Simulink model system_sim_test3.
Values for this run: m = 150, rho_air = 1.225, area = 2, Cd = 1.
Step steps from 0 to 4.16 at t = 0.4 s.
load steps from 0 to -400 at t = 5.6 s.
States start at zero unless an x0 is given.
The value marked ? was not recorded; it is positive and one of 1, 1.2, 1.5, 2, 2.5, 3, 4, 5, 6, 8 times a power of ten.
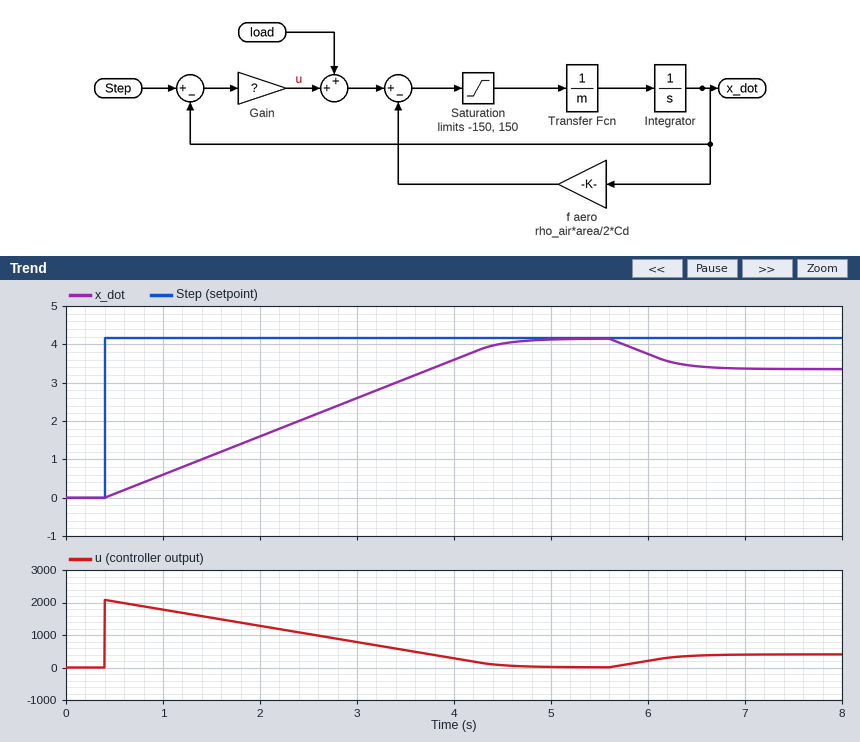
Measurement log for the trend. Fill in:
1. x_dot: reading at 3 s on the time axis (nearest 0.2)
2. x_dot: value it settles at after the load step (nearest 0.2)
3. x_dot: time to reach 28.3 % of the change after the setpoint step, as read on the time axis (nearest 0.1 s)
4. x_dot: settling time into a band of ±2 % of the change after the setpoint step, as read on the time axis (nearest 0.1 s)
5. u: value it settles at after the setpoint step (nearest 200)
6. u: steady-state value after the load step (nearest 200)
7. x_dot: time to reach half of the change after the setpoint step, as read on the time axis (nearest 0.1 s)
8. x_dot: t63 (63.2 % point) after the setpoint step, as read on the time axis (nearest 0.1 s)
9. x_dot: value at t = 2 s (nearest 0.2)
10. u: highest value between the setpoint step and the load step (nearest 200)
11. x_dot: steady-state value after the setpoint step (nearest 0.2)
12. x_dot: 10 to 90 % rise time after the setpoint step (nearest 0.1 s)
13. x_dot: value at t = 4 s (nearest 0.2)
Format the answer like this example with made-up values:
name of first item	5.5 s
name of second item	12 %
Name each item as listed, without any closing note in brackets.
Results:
x_dot: reading at 3 s on the time axis	2.6
x_dot: value it settles at after the load step	3.4
x_dot: time to reach 28.3 % of the change after the setpoint step, as read on the time axis	1.6 s
x_dot: settling time into a band of ±2 % of the change after the setpoint step, as read on the time axis	4.6 s
u: value it settles at after the setpoint step	0
u: steady-state value after the load step	400
x_dot: time to reach half of the change after the setpoint step, as read on the time axis	2.5 s
x_dot: t63 (63.2 % point) after the setpoint step, as read on the time axis	3.0 s
x_dot: value at t = 2 s	1.6
u: highest value between the setpoint step and the load step	2000
x_dot: steady-state value after the setpoint step	4.2
x_dot: 10 to 90 % rise time after the setpoint step	3.3 s
x_dot: value at t = 4 s	3.6
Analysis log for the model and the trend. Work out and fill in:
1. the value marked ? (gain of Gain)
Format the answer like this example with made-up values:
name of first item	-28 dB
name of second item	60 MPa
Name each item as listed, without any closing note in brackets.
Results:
the value marked ?	500
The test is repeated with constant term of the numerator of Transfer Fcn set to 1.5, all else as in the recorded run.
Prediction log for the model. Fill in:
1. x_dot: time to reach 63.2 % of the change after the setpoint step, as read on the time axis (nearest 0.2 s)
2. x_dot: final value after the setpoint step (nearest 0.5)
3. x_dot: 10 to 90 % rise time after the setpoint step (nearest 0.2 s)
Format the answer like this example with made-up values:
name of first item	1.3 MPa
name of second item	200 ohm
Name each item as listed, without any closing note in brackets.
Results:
x_dot: time to reach 63.2 % of the change after the setpoint step, as read on the time axis	2.2 s
x_dot: final value after the setpoint step	4.0
x_dot: 10 to 90 % rise time after the setpoint step	2.2 s
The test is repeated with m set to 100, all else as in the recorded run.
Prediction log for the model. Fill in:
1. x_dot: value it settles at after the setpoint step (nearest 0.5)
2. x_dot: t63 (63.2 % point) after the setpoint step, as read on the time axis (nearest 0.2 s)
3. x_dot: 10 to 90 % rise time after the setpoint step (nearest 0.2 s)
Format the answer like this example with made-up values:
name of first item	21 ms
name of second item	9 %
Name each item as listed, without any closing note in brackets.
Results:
x_dot: value it settles at after the setpoint step	4.0
x_dot: t63 (63.2 % point) after the setpoint step, as read on the time axis	2.2 s
x_dot: 10 to 90 % rise time after the setpoint step	2.2 s
